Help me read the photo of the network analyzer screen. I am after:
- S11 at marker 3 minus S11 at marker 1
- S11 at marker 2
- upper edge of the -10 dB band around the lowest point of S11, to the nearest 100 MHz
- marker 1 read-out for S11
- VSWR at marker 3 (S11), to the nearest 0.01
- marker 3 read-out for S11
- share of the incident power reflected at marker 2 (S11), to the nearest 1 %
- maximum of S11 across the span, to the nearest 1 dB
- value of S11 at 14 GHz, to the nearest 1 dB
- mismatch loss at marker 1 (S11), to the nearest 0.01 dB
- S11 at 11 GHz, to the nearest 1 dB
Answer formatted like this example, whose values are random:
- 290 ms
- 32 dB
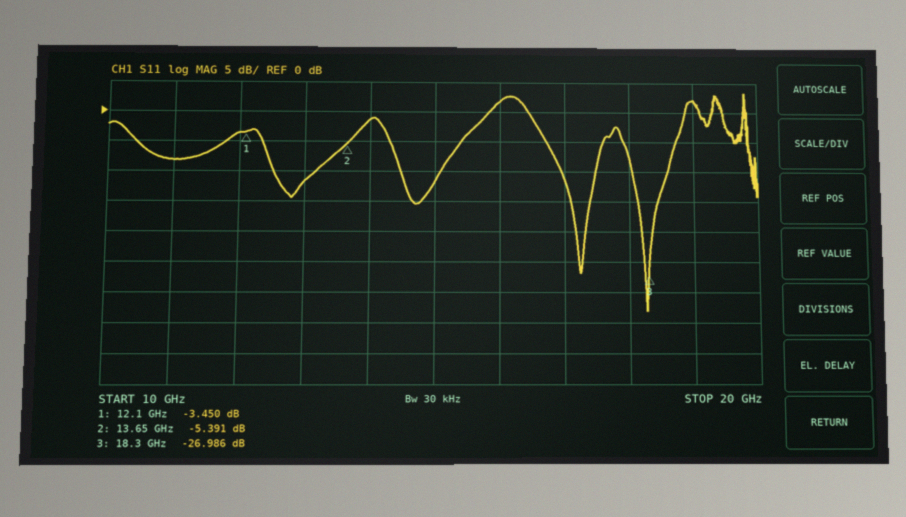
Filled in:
- -23.536 dB
- -5.391 dB
- 18.6 GHz
- -3.450 dB
- 1.09
- -26.986 dB
- 29 %
- 3 dB
- -1 dB
- 2.61 dB
- -8 dB
